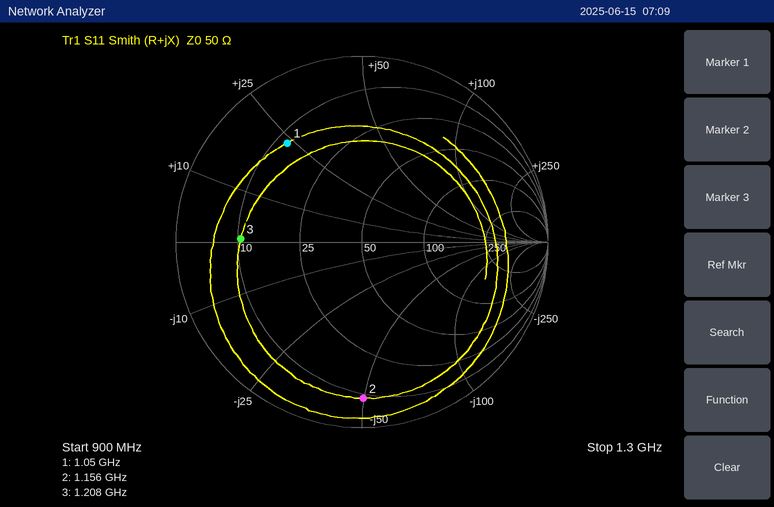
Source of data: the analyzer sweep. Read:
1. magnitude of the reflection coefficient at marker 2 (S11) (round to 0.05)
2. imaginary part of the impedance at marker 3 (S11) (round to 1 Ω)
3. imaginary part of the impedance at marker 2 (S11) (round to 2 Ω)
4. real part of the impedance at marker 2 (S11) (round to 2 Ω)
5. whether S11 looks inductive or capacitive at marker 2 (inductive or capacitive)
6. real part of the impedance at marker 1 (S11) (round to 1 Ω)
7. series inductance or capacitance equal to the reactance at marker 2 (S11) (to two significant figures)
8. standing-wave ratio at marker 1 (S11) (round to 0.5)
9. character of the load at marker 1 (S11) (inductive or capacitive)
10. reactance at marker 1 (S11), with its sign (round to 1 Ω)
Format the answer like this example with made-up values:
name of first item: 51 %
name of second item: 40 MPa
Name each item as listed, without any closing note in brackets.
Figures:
magnitude of the reflection coefficient at marker 2 (S11): 0.85
imaginary part of the impedance at marker 3 (S11): +1 Ω
imaginary part of the impedance at marker 2 (S11): -50 Ω
real part of the impedance at marker 2 (S11): 8 Ω
whether S11 looks inductive or capacitive at marker 2: capacitive
real part of the impedance at marker 1 (S11): 12 Ω
series inductance or capacitance equal to the reactance at marker 2 (S11): 2.8 pF
standing-wave ratio at marker 1 (S11): 5.0
character of the load at marker 1 (S11): inductive
reactance at marker 1 (S11), with its sign: +24 Ω
